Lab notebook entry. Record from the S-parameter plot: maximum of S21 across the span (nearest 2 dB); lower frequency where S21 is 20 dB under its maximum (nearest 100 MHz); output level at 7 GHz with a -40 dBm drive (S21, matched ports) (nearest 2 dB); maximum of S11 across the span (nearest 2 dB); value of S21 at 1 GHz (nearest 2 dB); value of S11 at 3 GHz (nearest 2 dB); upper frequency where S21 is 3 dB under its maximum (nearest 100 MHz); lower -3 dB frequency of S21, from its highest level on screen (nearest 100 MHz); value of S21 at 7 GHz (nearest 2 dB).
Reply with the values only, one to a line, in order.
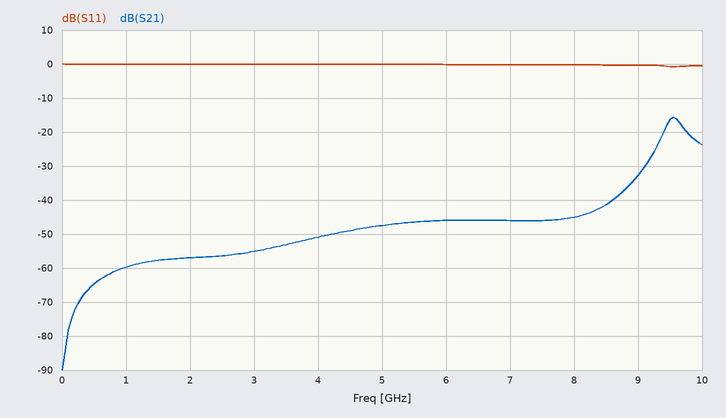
-16 dB
8.9 GHz
-86 dBm
0 dB
-60 dB
0 dB
9.7 GHz
9.4 GHz
-46 dB
